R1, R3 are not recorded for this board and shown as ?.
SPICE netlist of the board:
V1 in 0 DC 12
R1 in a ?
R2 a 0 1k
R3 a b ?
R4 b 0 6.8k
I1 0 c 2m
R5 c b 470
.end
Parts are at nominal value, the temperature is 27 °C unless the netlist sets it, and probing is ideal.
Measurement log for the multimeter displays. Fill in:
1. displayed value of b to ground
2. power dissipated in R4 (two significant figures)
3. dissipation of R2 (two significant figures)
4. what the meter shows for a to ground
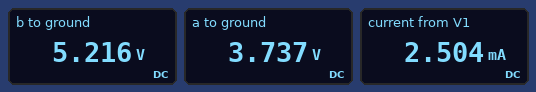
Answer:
5.216 V
4.0 mW
14 mW
3.737 V
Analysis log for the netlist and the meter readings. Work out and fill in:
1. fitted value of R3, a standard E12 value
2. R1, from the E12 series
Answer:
1.2 kΩ
3.3 kΩ
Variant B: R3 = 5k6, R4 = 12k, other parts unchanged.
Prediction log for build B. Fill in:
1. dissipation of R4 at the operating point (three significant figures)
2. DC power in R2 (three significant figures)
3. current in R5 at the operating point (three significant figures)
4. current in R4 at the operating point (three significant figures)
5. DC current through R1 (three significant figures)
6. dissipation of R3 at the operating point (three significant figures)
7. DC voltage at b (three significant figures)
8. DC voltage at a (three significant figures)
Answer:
8.57 mW
13.5 mW
2.00 mA
845 µA
2.52 mA
7.47 mW
10.1 V
3.68 V
